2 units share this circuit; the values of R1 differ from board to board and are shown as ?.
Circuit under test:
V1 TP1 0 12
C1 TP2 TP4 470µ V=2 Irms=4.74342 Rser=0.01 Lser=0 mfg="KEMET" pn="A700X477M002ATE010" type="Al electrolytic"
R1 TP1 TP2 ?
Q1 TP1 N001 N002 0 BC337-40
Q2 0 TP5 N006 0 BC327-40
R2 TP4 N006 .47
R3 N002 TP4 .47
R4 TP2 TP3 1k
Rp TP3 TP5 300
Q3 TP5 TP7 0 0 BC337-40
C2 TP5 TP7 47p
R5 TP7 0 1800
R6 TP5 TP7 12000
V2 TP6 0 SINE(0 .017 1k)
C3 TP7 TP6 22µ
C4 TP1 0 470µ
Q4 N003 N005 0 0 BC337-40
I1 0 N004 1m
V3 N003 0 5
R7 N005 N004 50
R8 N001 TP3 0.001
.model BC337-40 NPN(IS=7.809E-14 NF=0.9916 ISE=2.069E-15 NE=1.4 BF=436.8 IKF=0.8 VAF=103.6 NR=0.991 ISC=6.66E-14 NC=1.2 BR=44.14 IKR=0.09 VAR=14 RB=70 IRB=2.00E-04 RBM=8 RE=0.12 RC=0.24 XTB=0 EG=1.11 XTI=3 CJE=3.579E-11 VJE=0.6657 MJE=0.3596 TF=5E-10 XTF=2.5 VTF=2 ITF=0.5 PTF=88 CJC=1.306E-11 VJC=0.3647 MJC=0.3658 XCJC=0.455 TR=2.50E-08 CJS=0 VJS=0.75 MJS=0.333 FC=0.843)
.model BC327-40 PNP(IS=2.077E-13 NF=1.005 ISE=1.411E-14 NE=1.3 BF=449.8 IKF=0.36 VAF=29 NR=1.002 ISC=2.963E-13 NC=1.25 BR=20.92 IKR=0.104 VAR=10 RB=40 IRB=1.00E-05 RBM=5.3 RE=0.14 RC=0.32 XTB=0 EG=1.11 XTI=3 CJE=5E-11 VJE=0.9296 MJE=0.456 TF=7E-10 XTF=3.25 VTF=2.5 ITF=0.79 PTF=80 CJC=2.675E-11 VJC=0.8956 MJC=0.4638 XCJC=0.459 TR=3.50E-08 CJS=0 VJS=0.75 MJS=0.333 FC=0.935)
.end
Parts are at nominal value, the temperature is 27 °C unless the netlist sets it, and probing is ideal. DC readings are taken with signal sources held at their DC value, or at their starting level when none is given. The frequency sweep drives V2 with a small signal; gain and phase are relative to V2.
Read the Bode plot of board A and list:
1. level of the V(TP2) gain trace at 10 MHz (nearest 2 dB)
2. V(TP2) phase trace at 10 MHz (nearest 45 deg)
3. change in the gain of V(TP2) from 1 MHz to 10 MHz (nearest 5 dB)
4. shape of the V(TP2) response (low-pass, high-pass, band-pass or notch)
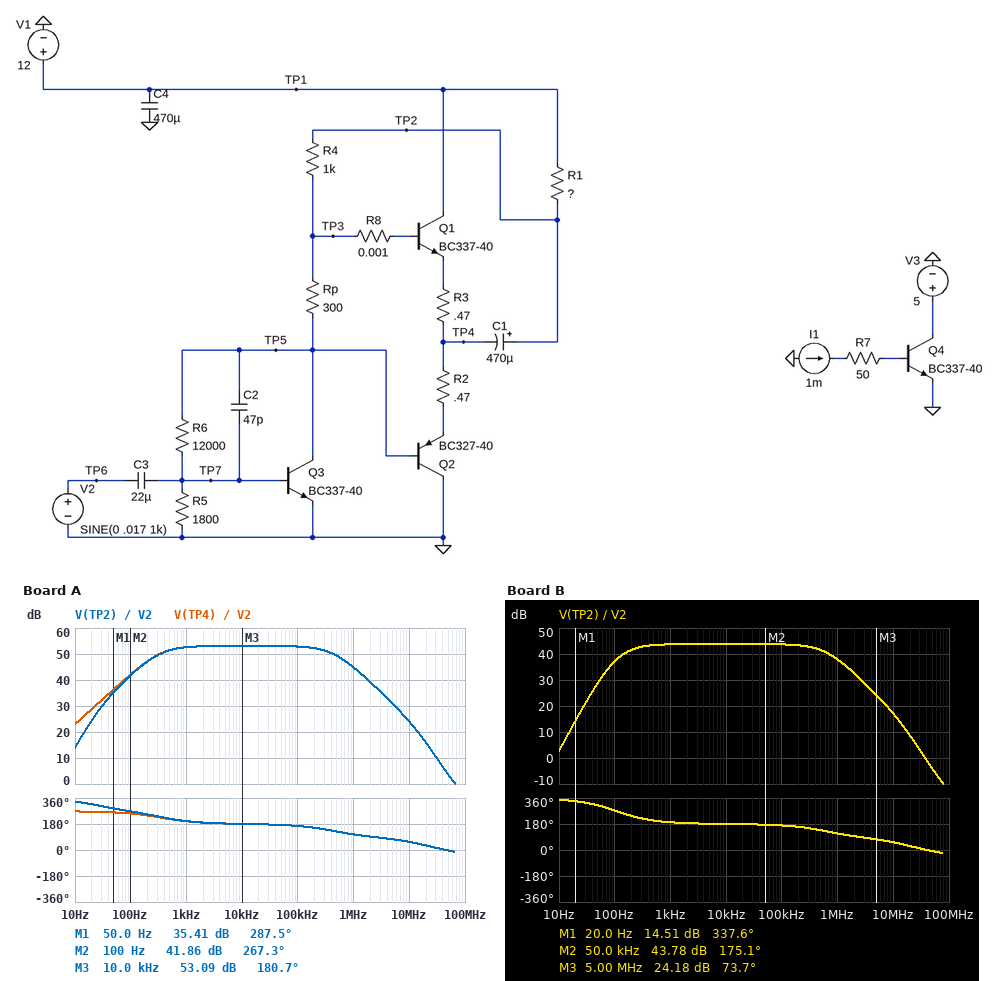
24 dB
45 deg
-20 dB
band-pass
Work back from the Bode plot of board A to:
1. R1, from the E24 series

13 Ω
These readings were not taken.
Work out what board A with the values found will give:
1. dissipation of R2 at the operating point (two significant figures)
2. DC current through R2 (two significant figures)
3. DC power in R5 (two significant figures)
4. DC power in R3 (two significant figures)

3.9 mW
91 mA
230 µW
3.9 mW
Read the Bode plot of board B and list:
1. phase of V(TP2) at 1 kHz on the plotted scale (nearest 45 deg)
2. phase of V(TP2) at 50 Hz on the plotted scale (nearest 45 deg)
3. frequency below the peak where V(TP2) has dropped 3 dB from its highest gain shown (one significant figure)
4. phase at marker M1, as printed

180 deg
315 deg
200 Hz
337.6 deg
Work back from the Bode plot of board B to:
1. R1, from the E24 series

3.3 Ω
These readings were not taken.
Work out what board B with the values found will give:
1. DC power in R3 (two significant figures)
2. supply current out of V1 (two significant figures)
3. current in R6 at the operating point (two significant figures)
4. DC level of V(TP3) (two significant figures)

4.3 mW
100 mA
370 µA
6.6 V
